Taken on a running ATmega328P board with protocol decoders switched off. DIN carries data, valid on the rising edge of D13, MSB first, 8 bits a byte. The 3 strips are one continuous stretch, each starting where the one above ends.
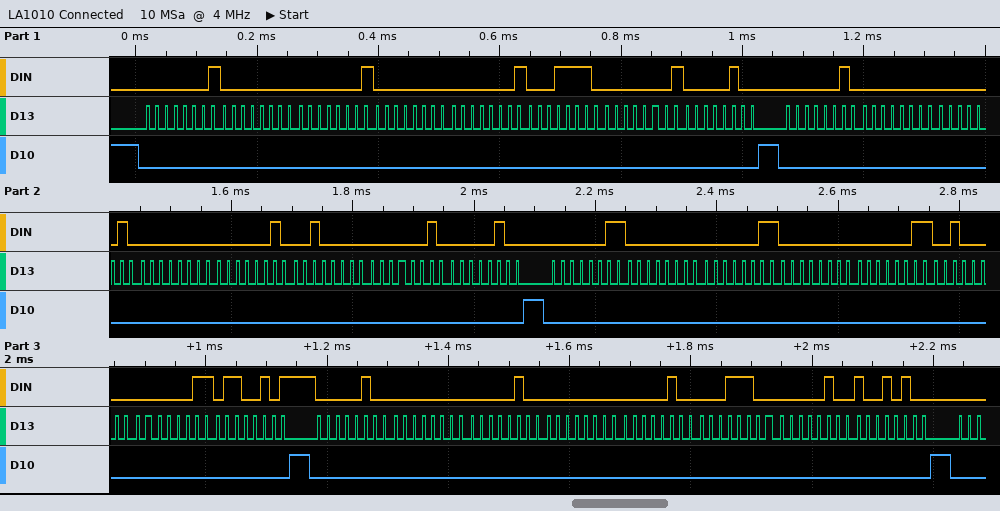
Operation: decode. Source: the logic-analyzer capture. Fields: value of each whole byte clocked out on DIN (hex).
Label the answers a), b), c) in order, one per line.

a) 01 00 01 00 01 1E 01 04 02 00 02 00 02 20 02 04 03 00 03 00 03 20 03 65 04 00 04 00 04 1C 04 94
